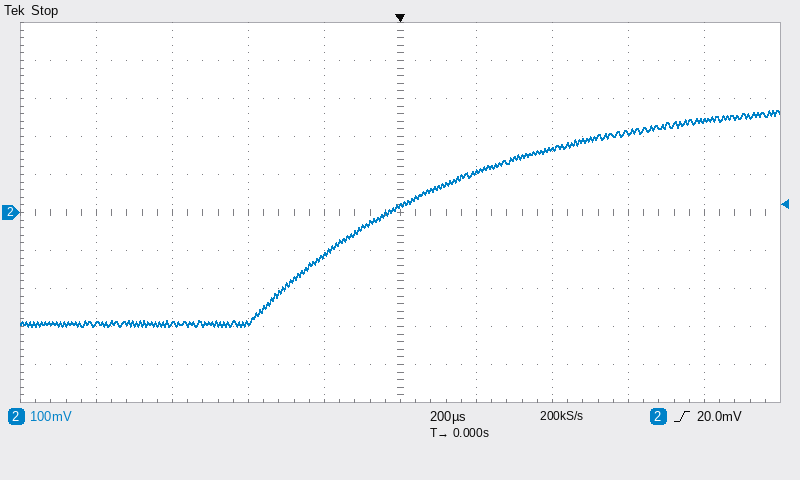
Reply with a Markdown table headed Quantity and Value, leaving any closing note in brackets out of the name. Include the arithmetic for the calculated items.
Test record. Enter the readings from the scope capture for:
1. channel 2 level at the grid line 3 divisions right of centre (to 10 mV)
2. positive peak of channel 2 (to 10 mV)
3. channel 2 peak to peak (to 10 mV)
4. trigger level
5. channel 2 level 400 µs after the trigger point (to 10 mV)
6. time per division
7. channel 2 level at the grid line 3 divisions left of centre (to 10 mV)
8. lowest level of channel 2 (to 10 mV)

| Quantity | Value |
|---|---|
| channel 2 level at the grid line 3 divisions right of centre | 210 mV |
| positive peak of channel 2 | 270 mV |
| channel 2 peak to peak | 270 mV − (-300 mV) = 570 mV |
| trigger level | 20.0 mV |
| channel 2 level 400 µs after the trigger point | 170 mV |
| time per division | 200 µs |
| channel 2 level at the grid line 3 divisions left of centre | -290 mV |
| lowest level of channel 2 | -300 mV |
